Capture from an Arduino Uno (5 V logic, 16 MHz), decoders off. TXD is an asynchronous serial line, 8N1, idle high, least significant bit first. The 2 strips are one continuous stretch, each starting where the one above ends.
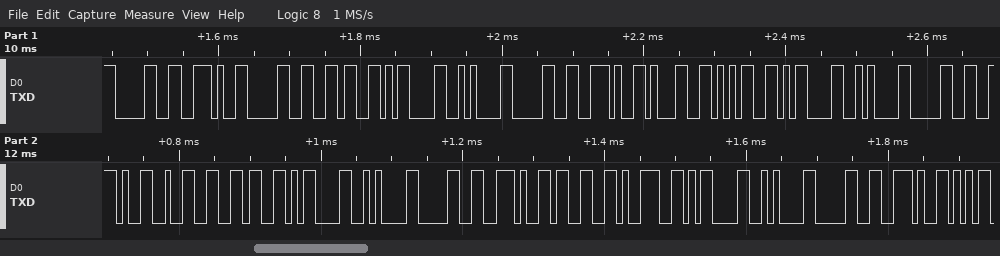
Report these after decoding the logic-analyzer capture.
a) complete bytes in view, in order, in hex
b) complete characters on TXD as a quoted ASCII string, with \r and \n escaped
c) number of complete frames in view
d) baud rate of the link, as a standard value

0x30 0x2E 0x30 0x36 0x0D 0x0A 0x30 0x2E 0x31 0x35 0x0D 0x0A 0x30 0x2E 0x32 0x36 0x0D 0x0A 0x30 0x2E 0x33 0x39 0x0D 0x0A 0x30 0x2E
"0.06\r\n0.15\r\n0.26\r\n0.39\r\n0."
26
115200 baud
